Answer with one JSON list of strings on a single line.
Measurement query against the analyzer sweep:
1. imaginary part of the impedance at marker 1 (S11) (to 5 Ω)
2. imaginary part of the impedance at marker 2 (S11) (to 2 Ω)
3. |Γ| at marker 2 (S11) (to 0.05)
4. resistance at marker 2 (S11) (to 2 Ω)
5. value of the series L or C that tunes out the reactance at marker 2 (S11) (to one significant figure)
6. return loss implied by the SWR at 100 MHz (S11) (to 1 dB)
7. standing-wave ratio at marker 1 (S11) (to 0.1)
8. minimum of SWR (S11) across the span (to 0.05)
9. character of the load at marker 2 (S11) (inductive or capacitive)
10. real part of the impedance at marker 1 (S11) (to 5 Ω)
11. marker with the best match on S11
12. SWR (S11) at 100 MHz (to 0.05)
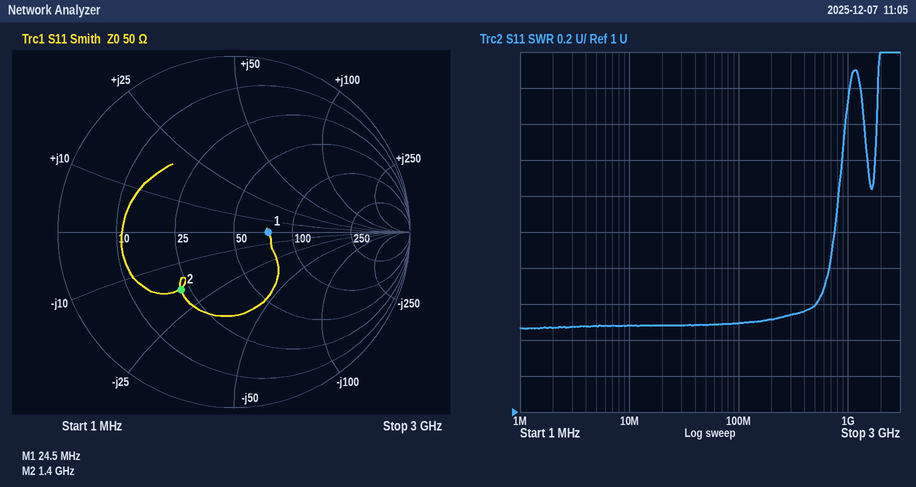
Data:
["0 Ω", "-18 Ω", "0.45", "22 Ω", "2 nH", "14 dB", "1.5", "1.45", "capacitive", "75 Ω", "marker 1", "1.50"]
